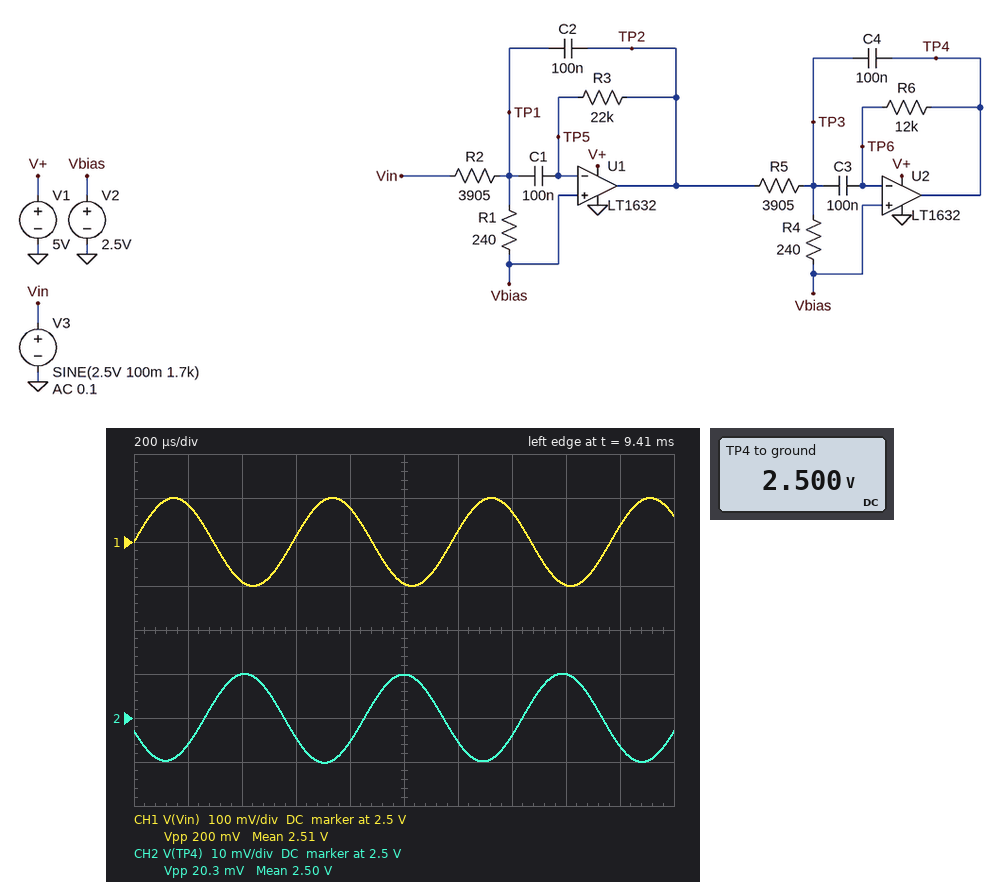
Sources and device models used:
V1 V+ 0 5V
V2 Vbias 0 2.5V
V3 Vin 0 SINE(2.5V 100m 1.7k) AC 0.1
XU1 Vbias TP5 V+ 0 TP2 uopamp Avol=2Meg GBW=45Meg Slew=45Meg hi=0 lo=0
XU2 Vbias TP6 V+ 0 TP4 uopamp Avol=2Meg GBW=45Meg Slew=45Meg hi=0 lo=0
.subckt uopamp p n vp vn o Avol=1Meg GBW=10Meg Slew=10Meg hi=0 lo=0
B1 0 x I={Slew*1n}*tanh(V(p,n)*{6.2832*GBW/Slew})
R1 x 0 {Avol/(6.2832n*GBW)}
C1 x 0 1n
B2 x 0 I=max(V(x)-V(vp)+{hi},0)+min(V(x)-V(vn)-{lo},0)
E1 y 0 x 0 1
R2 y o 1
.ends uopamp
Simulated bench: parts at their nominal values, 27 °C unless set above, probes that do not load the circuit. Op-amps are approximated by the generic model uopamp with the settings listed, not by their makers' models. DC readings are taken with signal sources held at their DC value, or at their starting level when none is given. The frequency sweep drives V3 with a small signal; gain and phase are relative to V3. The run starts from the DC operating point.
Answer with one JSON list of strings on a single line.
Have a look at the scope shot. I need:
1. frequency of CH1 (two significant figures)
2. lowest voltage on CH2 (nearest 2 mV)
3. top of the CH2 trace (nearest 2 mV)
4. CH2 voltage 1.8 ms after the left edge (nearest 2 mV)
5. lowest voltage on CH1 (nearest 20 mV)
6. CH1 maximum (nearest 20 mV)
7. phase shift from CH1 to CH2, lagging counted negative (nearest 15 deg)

["1.7 kHz", "2.490 V", "2.510 V", "2.494 V", "2.40 V", "2.60 V", "-165 deg"]
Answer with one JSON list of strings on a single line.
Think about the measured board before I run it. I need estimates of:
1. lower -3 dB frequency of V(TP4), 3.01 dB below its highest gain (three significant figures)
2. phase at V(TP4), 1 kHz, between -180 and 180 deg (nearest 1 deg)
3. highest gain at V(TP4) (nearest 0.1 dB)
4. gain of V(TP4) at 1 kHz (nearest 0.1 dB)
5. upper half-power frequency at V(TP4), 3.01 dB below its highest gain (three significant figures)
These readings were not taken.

["673 Hz", "-88 deg", "5.3 dB", "1.5 dB", "977 Hz"]
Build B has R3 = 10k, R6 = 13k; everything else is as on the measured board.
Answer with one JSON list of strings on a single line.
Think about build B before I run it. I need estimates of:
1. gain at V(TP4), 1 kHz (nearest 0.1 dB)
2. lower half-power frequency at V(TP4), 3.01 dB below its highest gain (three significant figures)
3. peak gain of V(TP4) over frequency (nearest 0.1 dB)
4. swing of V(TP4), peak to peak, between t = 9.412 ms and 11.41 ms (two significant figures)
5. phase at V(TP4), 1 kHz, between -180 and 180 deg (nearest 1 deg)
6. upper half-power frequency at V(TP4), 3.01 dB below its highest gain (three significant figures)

["4.8 dB", "880 Hz", "4.9 dB", "25 mV", "-9 deg", "1.10 kHz"]
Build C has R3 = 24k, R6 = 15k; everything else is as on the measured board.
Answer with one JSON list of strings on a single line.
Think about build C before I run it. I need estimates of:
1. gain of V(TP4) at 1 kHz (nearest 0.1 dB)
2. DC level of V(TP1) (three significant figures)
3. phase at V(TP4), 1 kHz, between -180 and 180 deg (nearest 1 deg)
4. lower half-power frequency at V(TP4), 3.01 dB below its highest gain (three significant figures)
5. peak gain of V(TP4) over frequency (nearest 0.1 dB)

["-0.8 dB", "2.50 V", "-126 deg", "650 Hz", "9.2 dB"]
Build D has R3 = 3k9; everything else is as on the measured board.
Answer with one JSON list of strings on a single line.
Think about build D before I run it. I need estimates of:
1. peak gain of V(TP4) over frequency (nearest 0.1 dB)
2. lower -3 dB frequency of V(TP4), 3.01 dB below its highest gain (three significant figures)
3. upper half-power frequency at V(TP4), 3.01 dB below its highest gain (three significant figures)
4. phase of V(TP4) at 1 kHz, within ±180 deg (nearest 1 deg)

["-10.5 dB", "884 Hz", "1.32 kHz", "52 deg"]
